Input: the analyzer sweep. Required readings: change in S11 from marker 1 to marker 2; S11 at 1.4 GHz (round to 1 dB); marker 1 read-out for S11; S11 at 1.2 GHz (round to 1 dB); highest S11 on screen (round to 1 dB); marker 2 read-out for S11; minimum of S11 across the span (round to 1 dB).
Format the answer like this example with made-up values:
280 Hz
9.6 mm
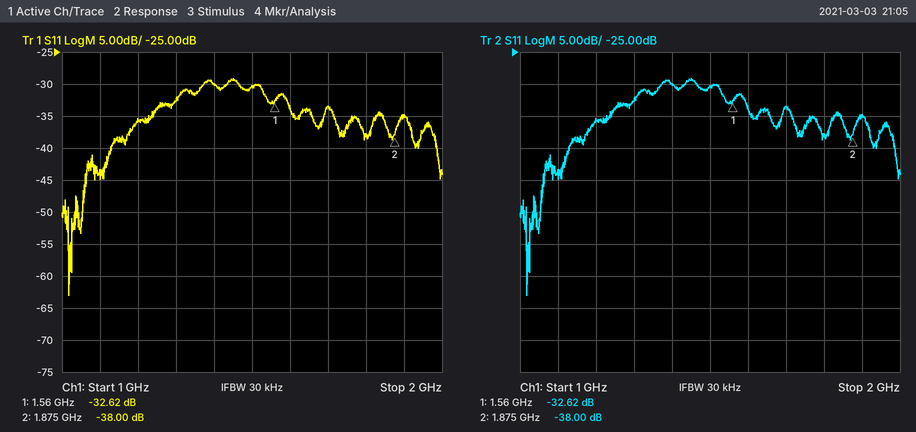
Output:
-5.38 dB
-30 dB
-32.62 dB
-36 dB
-29 dB
-38.00 dB
-63 dB
